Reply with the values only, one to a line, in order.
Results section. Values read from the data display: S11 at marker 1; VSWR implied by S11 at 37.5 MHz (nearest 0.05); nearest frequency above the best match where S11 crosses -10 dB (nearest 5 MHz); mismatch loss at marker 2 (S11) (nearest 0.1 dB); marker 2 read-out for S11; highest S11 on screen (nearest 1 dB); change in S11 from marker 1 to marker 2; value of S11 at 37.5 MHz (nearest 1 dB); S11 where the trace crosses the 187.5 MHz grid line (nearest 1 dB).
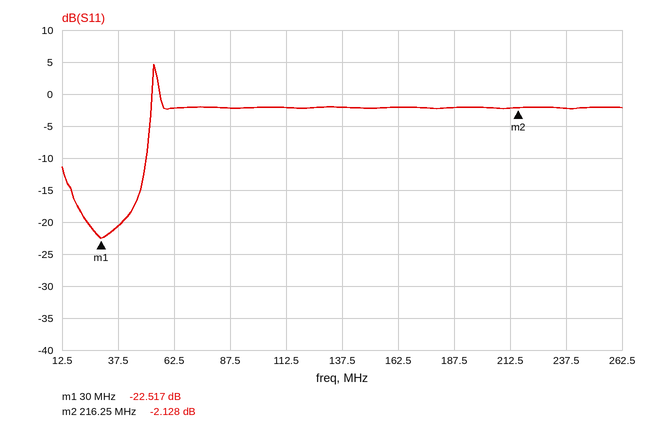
-22.517 dB
1.20
50 MHz
4.1 dB
-2.128 dB
5 dB
20.389 dB
-21 dB
-2 dB
